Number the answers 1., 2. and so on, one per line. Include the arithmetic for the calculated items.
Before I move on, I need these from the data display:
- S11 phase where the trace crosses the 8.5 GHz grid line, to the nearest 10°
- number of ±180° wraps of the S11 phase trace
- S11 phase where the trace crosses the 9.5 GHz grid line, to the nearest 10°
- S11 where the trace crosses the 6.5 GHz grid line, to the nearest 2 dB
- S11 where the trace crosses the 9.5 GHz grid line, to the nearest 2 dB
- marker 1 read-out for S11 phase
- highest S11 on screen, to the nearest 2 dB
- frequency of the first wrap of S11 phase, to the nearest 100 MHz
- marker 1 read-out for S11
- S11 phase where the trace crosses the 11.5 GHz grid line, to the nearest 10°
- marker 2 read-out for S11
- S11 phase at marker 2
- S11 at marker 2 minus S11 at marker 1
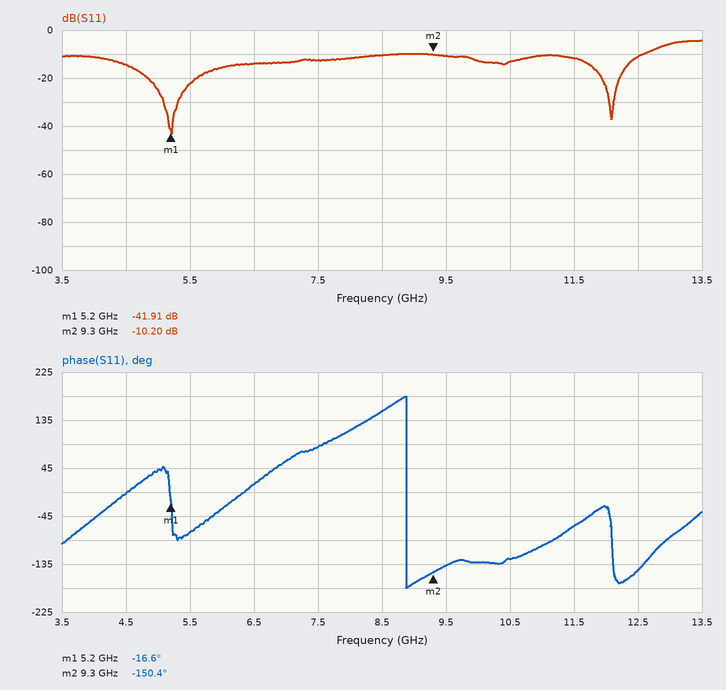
1. 150°
2. 1
3. -140°
4. -14 dB
5. -10 dB
6. -16.6°
7. -4 dB
8. 8.9 GHz
9. -41.91 dB
10. -60°
11. -10.20 dB
12. -150.4°
13. -10.2 − (-41.91) = 31.71 dB
